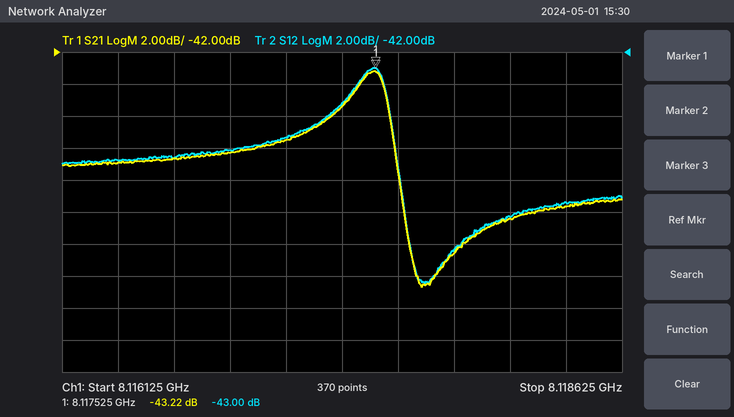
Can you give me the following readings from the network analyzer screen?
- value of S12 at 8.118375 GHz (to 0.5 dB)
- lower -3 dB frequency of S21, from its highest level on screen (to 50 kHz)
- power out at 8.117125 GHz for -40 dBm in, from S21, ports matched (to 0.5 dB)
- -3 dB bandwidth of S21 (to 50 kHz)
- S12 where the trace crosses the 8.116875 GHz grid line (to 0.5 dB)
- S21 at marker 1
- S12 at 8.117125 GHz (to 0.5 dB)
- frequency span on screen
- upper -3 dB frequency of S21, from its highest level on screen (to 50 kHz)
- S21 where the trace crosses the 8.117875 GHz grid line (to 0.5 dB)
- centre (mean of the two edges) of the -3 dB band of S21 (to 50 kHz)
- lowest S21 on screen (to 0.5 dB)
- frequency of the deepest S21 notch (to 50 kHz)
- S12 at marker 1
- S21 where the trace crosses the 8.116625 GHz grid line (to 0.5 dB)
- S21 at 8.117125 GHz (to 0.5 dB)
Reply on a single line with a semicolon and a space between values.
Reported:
-51.5 dB; 8.11730 GHz; -87.5 dBm; 300 kHz; -48.0 dB; -43.22 dB; -47.5 dB; 2.5 MHz; 8.11760 GHz; -54.5 dB; 8.11745 GHz; -56.5 dB; 8.11775 GHz; -43.00 dB; -48.5 dB; -47.5 dB
